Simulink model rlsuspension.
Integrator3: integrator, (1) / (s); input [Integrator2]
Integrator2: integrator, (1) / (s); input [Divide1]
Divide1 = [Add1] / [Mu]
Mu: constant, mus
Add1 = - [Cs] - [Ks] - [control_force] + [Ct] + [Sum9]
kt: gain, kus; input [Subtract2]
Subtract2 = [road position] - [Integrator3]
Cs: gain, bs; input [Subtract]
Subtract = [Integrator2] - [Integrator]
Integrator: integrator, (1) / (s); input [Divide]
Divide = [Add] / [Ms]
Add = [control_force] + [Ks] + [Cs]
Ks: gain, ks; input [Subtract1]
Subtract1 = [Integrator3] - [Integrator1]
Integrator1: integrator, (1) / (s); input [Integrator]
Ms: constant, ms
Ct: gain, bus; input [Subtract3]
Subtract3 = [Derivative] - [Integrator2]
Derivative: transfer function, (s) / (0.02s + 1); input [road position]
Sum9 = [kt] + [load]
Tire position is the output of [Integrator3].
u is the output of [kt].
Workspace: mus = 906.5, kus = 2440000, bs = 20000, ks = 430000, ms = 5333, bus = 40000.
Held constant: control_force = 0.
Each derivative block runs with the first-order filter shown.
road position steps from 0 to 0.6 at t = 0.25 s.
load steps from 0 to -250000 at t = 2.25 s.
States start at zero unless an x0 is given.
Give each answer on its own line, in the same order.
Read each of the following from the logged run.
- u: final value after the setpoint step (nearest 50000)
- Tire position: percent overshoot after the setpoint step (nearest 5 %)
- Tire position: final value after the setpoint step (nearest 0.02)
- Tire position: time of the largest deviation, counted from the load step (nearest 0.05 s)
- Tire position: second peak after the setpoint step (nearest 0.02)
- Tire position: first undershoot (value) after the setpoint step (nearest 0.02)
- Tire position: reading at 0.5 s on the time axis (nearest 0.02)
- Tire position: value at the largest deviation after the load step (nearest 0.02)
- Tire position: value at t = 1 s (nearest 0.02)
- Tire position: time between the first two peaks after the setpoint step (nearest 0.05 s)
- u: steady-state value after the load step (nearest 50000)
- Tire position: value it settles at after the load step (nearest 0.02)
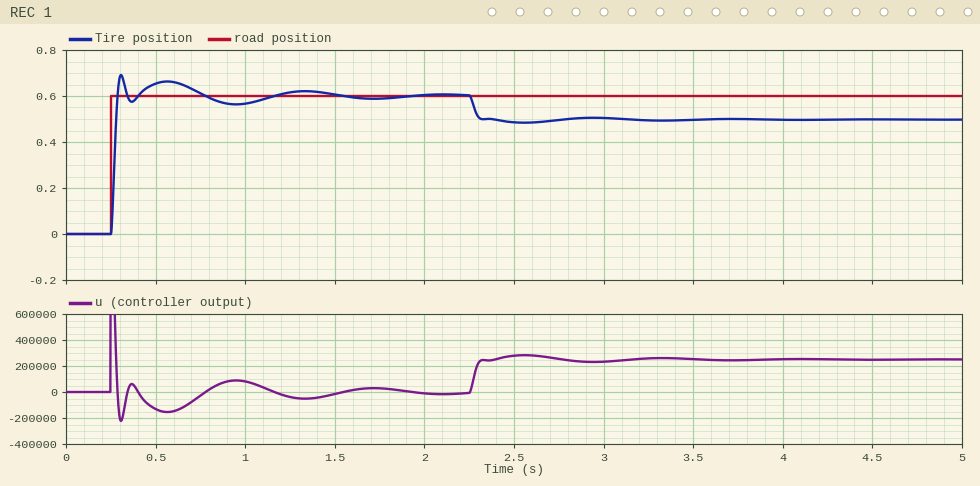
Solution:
0
15 %
0.60
0.30 s
0.66
0.58
0.66
0.48
0.56
0.25 s
250000
0.50
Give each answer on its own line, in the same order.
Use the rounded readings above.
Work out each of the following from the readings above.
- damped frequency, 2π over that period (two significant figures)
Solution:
25 rad/s
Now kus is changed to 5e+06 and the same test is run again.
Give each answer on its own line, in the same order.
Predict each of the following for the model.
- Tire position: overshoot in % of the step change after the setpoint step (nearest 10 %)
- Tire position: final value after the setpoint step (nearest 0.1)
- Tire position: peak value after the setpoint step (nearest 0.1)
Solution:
30 %
0.6
0.8
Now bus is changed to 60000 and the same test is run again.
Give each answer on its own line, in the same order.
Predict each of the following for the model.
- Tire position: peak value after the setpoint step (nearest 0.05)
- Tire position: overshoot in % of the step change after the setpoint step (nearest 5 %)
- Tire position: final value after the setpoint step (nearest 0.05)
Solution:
0.65
10 %
0.60
